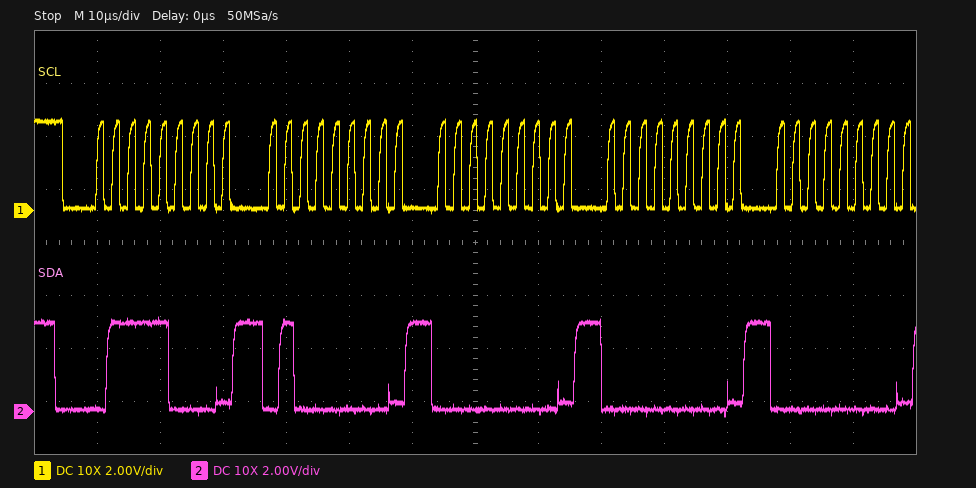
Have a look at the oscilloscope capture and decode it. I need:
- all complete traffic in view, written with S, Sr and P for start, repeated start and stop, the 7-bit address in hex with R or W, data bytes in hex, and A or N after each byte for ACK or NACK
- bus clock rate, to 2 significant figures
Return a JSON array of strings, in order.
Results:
["S 3CW A 40 A 00 A 00 A 00 A", "400 kHz"]
